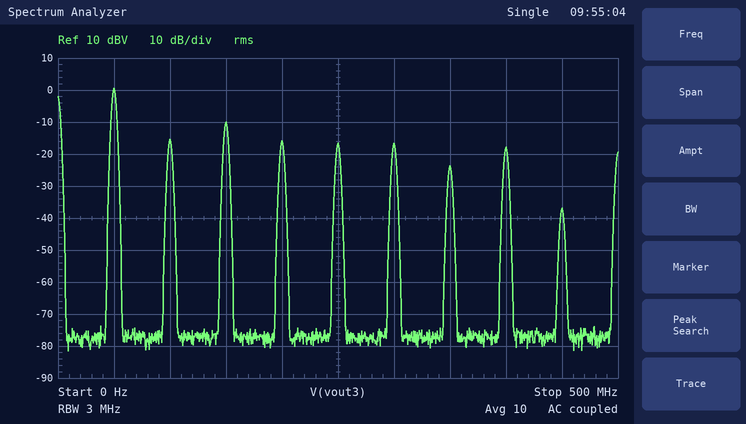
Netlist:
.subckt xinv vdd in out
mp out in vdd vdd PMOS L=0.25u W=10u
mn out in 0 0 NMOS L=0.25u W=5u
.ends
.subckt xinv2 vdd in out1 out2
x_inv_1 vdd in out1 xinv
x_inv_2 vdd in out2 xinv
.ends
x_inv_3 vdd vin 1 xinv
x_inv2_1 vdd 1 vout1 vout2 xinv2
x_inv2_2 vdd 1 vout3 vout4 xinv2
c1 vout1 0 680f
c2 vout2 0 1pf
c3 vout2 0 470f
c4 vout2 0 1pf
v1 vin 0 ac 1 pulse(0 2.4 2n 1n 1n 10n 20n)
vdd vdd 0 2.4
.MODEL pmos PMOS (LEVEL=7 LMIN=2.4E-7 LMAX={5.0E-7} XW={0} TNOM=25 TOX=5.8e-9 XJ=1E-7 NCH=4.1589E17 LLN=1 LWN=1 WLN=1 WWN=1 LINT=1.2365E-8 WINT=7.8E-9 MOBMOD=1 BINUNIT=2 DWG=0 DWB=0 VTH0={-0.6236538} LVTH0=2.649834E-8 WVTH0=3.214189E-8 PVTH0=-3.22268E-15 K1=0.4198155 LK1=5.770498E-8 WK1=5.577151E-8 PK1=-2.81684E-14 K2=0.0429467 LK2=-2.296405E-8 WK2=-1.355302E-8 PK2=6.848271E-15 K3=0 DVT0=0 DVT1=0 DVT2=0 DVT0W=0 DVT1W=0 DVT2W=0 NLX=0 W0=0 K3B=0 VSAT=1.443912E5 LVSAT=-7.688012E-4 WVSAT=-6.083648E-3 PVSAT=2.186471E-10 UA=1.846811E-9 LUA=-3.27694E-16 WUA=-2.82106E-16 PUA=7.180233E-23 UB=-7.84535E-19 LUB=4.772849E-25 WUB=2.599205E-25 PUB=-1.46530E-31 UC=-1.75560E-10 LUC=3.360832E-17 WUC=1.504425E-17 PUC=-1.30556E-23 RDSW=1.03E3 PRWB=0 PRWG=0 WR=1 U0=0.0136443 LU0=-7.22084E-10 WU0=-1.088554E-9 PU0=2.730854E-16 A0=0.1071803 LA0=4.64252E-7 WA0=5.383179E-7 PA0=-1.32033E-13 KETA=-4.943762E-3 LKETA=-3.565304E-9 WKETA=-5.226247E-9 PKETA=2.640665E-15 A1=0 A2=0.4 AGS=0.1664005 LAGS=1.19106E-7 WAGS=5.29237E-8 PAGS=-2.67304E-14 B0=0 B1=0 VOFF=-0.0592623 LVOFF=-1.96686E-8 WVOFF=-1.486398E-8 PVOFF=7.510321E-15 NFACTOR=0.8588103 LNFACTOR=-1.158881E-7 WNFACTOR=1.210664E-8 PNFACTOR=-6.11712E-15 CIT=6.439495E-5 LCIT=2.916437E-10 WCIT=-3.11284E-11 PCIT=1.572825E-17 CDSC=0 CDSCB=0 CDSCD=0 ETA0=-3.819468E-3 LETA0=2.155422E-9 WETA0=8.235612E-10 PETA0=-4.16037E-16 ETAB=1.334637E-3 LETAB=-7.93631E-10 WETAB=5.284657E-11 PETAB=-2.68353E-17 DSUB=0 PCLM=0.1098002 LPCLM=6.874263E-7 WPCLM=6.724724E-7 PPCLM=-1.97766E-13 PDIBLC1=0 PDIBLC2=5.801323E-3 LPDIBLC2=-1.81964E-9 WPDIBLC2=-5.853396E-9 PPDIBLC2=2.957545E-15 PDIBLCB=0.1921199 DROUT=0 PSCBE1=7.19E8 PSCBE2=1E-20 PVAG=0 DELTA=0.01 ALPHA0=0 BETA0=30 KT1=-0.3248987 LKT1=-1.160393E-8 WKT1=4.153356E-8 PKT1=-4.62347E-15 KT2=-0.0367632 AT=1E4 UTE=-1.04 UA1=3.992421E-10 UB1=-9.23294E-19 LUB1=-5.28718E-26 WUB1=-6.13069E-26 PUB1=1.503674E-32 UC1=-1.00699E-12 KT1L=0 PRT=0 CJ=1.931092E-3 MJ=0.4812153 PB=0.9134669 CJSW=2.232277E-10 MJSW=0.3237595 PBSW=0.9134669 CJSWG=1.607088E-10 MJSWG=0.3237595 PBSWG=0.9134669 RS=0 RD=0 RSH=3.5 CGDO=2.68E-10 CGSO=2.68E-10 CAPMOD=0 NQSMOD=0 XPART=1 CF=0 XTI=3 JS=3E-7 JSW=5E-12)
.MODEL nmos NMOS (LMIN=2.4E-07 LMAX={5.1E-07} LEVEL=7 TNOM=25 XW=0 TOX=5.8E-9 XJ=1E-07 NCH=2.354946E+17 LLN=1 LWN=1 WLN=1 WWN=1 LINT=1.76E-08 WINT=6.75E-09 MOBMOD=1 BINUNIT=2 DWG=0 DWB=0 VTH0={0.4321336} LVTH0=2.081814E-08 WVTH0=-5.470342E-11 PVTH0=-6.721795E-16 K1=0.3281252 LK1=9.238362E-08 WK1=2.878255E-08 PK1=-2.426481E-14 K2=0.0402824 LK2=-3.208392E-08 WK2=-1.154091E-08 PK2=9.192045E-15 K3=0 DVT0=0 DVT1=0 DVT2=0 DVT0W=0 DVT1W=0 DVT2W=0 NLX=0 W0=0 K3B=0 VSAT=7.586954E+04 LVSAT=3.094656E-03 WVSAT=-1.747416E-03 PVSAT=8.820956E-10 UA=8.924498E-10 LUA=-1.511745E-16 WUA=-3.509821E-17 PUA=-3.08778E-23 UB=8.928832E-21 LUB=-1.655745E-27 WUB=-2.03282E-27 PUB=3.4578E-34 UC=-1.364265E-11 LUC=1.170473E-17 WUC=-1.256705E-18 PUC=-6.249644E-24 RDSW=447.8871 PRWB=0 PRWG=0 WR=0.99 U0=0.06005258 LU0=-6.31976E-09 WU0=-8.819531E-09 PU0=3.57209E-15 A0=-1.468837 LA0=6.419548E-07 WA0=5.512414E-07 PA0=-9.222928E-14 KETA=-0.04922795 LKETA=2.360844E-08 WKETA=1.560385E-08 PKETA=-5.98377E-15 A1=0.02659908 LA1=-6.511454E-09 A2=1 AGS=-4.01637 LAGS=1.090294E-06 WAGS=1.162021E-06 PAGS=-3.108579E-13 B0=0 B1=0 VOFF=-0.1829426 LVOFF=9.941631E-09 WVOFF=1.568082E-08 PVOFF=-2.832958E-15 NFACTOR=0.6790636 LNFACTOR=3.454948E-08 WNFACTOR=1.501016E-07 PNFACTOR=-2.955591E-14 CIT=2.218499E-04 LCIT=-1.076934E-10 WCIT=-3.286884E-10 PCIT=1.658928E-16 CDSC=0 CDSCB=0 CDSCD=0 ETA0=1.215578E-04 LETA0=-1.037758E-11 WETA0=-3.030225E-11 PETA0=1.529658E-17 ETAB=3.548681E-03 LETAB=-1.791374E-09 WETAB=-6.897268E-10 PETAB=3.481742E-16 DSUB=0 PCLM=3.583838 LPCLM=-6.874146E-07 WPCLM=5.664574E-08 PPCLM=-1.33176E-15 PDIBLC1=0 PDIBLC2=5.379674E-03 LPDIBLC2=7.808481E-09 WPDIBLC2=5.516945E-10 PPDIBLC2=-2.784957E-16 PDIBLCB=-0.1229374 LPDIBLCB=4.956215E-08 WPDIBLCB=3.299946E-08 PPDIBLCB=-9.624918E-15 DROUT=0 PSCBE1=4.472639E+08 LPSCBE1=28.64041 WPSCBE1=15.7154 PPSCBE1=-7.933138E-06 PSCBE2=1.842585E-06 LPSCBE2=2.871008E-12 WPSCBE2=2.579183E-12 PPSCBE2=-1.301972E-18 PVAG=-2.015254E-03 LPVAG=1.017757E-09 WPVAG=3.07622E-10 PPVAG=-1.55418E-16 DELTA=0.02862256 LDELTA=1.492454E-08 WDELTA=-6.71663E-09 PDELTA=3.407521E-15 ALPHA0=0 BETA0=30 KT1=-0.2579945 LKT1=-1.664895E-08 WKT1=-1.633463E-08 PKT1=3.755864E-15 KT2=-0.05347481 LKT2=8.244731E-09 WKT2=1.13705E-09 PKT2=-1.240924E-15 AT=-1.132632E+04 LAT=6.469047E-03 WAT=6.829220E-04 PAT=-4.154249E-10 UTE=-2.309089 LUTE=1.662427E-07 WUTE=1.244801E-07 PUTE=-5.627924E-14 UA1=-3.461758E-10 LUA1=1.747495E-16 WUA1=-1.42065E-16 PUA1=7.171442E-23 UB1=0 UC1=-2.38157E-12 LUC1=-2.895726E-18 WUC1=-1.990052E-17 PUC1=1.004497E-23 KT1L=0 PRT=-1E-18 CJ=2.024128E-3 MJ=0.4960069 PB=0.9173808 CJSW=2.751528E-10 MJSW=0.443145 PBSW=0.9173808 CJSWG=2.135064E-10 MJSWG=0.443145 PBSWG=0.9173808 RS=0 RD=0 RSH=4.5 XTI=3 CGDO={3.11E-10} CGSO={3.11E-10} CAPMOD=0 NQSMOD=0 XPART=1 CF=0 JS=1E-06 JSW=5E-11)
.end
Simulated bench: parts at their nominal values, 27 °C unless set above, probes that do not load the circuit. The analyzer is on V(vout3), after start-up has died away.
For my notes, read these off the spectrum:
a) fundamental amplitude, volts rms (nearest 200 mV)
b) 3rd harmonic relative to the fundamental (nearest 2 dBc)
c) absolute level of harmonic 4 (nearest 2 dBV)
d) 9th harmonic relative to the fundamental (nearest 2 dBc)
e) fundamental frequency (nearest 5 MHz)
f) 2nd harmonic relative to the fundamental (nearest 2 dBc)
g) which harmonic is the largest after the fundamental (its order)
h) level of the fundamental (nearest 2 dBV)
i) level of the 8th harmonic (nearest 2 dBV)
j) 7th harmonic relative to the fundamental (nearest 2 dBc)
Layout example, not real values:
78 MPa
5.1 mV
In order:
1.0 V
-10 dBc
-16 dBV
-38 dBc
50 MHz
-16 dBc
3
0 dBV
-18 dBV
-24 dBc
